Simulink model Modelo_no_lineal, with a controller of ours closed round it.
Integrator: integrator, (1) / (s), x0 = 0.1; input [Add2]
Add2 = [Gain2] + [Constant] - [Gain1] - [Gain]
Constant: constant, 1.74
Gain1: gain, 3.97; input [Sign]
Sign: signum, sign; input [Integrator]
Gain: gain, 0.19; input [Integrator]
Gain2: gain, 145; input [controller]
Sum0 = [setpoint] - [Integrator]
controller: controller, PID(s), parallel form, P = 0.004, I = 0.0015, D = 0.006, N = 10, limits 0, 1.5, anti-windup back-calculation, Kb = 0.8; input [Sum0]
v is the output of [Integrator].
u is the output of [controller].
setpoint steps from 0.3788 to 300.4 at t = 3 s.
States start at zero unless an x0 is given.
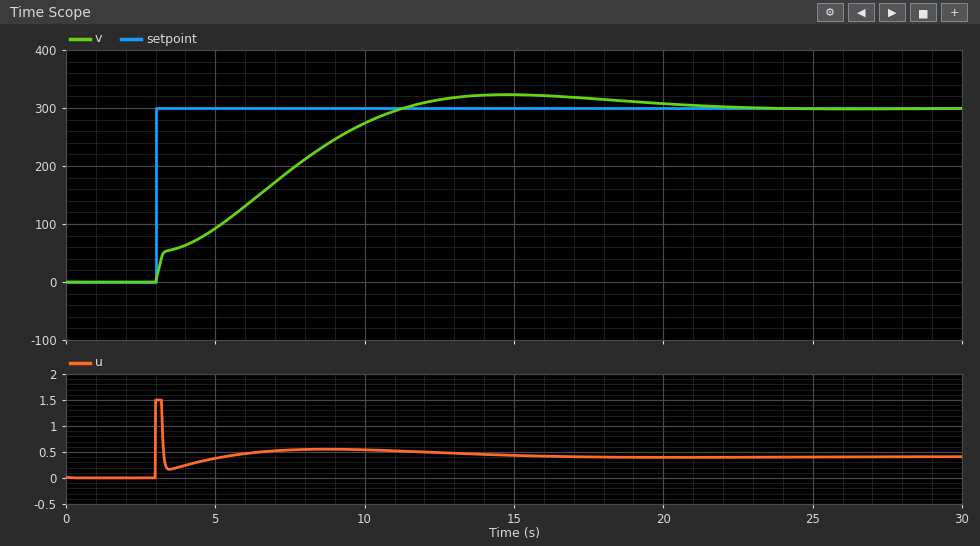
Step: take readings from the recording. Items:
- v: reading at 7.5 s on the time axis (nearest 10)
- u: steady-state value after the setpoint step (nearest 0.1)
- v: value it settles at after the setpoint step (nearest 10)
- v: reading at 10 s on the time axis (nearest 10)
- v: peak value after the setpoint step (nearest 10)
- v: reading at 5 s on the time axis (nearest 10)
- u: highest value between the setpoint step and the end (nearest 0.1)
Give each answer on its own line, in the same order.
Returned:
190
0.4
300
270
320
90
1.5
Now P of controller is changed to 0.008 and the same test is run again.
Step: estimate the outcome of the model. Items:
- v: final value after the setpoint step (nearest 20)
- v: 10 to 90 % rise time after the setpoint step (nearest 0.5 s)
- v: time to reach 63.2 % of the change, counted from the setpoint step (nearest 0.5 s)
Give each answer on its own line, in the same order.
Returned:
300
8.5 s
3.5 s
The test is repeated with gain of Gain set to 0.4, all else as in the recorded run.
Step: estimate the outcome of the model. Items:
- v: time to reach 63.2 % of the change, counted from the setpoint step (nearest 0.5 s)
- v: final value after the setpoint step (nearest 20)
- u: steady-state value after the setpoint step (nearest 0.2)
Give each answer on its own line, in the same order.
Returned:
5.0 s
300
0.8
